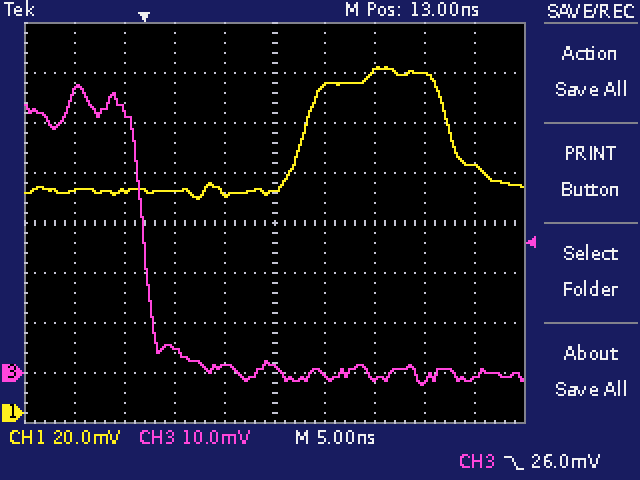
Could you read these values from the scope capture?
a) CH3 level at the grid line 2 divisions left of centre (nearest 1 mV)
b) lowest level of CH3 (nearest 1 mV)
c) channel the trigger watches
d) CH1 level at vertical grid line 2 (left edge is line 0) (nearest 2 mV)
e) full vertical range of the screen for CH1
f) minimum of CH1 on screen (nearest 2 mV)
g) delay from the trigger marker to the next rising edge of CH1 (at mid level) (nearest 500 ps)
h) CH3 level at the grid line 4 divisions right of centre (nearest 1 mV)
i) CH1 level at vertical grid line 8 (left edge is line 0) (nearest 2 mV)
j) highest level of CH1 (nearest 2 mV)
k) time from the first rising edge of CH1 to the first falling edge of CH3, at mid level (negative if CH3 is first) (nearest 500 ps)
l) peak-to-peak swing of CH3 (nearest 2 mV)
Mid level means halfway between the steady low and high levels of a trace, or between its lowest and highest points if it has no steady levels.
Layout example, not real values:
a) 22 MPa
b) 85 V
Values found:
a) 5 mV
b) -2 mV
c) CH3
d) 88 mV
e) 160 mV
f) 86 mV
g) 16.0 ns
h) -1 mV
i) 136 mV
j) 138 mV
k) -16.0 ns
l) 60 mV
